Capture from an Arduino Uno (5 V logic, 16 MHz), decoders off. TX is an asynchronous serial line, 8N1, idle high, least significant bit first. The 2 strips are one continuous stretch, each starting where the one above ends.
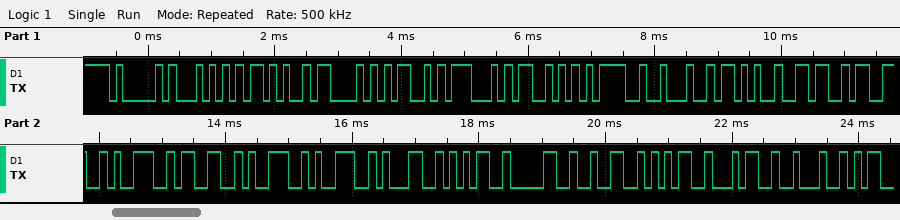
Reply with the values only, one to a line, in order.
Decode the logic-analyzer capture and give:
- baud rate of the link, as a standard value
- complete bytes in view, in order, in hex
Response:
9600 baud
41 54 2B 43 4D 47 53 3D 22 2B 36 33 39 33 39 39 31 35 30 32 35 34 22
